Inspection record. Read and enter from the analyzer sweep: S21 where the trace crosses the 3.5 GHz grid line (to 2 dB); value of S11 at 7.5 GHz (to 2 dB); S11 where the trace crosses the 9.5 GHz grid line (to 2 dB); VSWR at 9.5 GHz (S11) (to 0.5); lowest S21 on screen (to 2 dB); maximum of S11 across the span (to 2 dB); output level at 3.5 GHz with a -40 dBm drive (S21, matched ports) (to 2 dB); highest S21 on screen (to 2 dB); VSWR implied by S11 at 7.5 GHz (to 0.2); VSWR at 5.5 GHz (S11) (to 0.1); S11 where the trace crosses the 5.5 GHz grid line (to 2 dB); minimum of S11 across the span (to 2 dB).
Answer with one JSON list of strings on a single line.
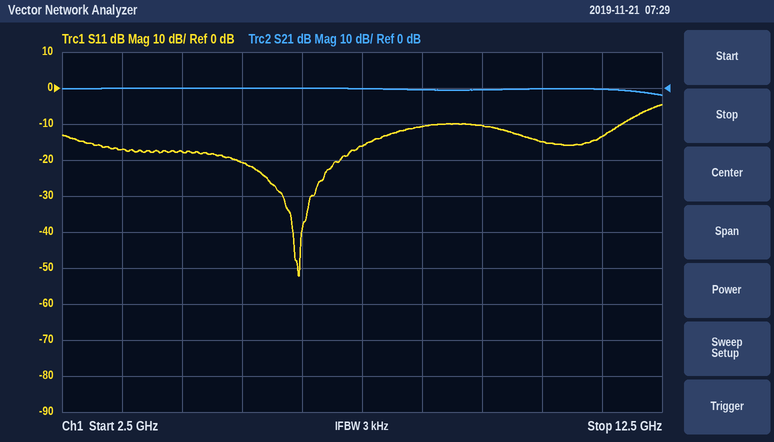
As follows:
["0 dB", "-16 dB", "-10 dB", "2.0", "-2 dB", "-4 dB", "-40 dBm", "0 dB", "1.4", "1.2", "-20 dB", "-52 dB"]
